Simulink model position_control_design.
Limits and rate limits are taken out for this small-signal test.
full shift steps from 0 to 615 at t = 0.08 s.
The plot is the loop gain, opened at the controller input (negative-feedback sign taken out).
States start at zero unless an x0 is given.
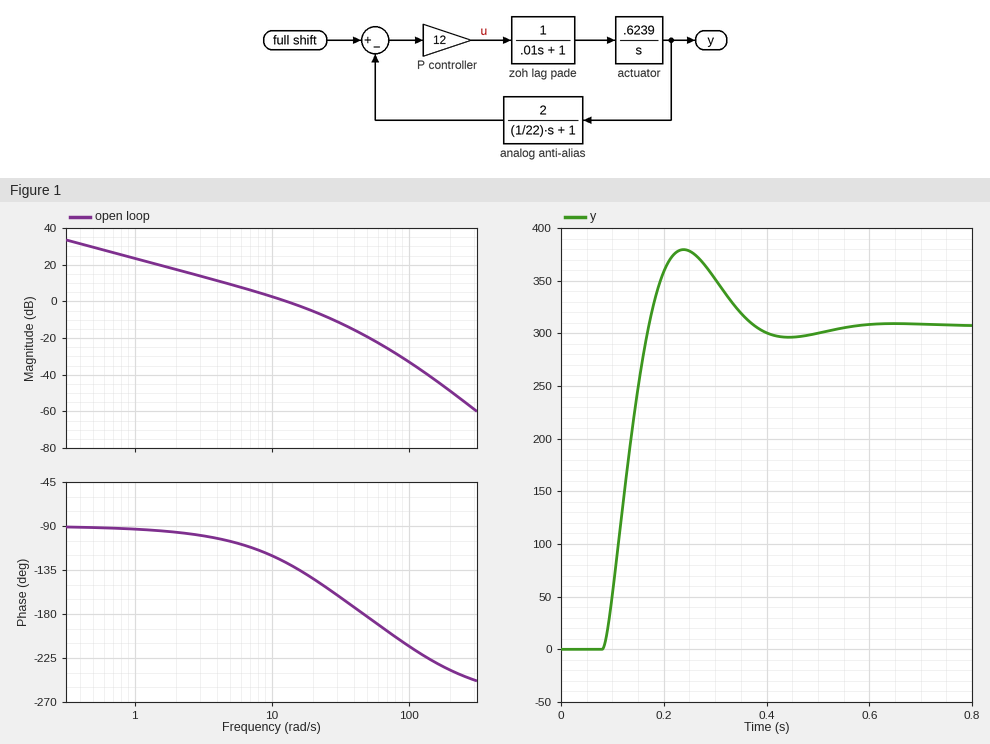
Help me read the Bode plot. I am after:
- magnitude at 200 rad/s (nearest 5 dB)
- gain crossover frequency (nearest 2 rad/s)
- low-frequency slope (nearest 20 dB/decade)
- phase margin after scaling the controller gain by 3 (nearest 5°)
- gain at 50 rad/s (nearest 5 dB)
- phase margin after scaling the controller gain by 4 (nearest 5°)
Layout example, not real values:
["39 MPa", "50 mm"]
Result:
["-50 dB", "12 rad/s", "-20 dB/decade", "25°", "-20 dB", "15°"]
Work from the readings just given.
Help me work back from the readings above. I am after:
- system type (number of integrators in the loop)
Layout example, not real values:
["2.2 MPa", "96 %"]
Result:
["1"]
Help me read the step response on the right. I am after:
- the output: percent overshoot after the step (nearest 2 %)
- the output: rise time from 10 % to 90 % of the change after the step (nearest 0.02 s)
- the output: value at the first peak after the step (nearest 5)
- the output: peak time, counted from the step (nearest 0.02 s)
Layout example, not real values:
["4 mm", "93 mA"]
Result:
["24 %", "0.06 s", "380", "0.16 s"]
